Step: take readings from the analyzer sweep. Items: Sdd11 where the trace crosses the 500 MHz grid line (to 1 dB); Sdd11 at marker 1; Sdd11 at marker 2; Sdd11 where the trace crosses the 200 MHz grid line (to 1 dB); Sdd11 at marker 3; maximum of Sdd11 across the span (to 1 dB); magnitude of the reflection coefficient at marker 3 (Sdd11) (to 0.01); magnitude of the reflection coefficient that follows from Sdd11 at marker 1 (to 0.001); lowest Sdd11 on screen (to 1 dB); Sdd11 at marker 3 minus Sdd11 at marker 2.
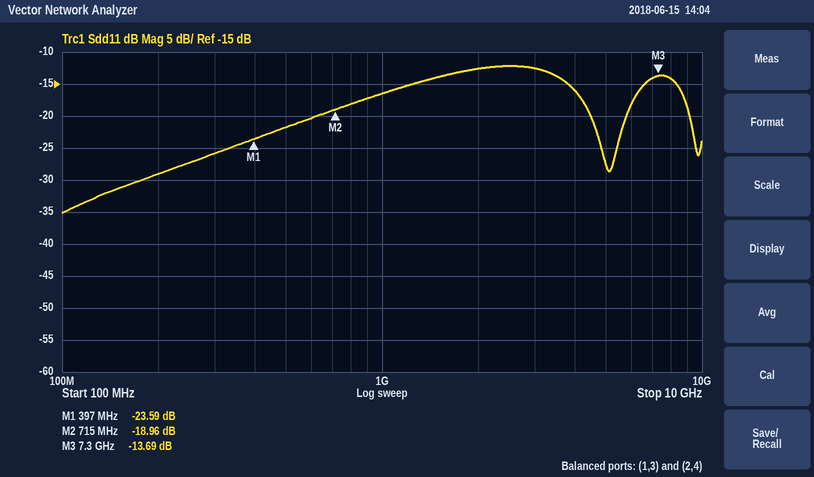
-22 dB
-23.59 dB
-18.96 dB
-29 dB
-13.69 dB
-12 dB
0.21
0.066
-35 dB
5.27 dB
